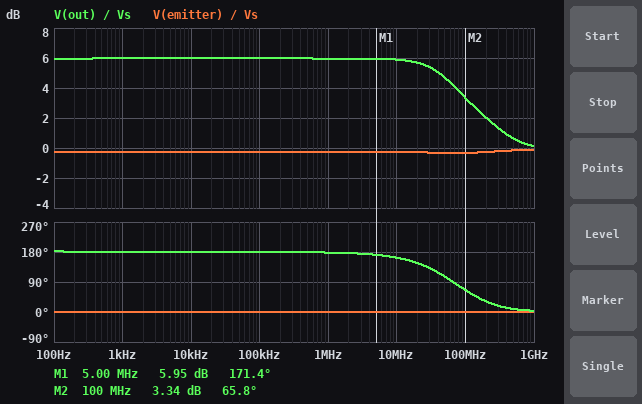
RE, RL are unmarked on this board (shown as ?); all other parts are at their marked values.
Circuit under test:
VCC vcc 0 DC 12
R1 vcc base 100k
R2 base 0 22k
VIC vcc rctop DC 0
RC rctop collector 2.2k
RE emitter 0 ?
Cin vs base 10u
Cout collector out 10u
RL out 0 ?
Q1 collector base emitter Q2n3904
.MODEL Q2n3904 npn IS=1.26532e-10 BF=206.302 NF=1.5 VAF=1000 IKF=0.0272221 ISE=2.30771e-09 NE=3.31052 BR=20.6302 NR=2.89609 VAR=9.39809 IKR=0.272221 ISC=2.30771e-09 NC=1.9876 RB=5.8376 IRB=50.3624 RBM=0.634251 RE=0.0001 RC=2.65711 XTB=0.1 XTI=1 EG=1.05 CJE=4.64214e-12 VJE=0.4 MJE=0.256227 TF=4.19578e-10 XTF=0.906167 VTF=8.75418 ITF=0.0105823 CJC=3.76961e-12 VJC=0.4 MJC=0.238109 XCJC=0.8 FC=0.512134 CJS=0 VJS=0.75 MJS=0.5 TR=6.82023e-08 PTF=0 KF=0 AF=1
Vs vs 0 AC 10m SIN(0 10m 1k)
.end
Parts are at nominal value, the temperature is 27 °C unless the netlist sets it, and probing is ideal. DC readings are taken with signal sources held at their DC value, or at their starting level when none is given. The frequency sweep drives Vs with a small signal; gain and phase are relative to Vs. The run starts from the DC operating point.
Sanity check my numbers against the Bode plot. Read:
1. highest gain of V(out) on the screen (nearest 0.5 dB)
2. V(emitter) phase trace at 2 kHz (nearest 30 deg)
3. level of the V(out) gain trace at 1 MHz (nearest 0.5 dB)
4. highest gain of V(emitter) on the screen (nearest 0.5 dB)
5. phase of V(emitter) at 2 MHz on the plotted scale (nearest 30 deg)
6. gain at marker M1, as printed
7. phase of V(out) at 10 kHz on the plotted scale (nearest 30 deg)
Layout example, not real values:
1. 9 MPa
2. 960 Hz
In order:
1. 6.0 dB
2. 0 deg
3. 6.0 dB
4. 0 dB
5. 0 deg
6. 5.95 dB
7. 180 deg
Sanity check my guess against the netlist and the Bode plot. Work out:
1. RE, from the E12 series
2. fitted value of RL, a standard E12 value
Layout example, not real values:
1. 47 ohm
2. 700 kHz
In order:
1. 680 Ω
2. 3.9 kΩ
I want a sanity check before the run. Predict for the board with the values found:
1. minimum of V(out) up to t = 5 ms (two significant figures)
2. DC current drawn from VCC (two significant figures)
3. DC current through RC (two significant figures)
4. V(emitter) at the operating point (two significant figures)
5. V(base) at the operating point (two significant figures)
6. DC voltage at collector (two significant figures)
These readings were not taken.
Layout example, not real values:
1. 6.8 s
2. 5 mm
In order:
1. -20 mV
2. 1.9 mA
3. 1.8 mA
4. 1.3 V
5. 1.9 V
6. 8.0 V
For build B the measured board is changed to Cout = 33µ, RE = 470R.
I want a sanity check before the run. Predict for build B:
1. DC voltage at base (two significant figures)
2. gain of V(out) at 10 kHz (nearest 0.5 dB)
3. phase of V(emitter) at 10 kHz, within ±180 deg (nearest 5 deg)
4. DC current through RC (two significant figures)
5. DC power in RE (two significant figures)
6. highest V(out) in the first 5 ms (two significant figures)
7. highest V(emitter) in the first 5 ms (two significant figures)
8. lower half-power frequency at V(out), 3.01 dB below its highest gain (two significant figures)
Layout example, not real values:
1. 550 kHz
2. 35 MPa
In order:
1. 1.8 V
2. 9.0 dB
3. 0 deg
4. 2.5 mA
5. 2.9 mW
6. 29 mV
7. 1.2 V
8. 1.5 Hz
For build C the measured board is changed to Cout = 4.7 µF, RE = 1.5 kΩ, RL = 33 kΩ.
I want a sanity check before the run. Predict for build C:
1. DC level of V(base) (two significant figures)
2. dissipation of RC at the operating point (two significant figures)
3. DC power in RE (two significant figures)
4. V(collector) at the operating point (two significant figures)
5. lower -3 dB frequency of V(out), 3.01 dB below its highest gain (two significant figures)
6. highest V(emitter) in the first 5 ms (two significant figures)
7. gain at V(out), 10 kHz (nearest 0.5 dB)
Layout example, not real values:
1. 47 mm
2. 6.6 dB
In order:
1. 2.0 V
2. 1.9 mW
3. 1.3 mW
4. 10 V
5. 1.5 Hz
6. 1.4 V
7. 2.5 dB
